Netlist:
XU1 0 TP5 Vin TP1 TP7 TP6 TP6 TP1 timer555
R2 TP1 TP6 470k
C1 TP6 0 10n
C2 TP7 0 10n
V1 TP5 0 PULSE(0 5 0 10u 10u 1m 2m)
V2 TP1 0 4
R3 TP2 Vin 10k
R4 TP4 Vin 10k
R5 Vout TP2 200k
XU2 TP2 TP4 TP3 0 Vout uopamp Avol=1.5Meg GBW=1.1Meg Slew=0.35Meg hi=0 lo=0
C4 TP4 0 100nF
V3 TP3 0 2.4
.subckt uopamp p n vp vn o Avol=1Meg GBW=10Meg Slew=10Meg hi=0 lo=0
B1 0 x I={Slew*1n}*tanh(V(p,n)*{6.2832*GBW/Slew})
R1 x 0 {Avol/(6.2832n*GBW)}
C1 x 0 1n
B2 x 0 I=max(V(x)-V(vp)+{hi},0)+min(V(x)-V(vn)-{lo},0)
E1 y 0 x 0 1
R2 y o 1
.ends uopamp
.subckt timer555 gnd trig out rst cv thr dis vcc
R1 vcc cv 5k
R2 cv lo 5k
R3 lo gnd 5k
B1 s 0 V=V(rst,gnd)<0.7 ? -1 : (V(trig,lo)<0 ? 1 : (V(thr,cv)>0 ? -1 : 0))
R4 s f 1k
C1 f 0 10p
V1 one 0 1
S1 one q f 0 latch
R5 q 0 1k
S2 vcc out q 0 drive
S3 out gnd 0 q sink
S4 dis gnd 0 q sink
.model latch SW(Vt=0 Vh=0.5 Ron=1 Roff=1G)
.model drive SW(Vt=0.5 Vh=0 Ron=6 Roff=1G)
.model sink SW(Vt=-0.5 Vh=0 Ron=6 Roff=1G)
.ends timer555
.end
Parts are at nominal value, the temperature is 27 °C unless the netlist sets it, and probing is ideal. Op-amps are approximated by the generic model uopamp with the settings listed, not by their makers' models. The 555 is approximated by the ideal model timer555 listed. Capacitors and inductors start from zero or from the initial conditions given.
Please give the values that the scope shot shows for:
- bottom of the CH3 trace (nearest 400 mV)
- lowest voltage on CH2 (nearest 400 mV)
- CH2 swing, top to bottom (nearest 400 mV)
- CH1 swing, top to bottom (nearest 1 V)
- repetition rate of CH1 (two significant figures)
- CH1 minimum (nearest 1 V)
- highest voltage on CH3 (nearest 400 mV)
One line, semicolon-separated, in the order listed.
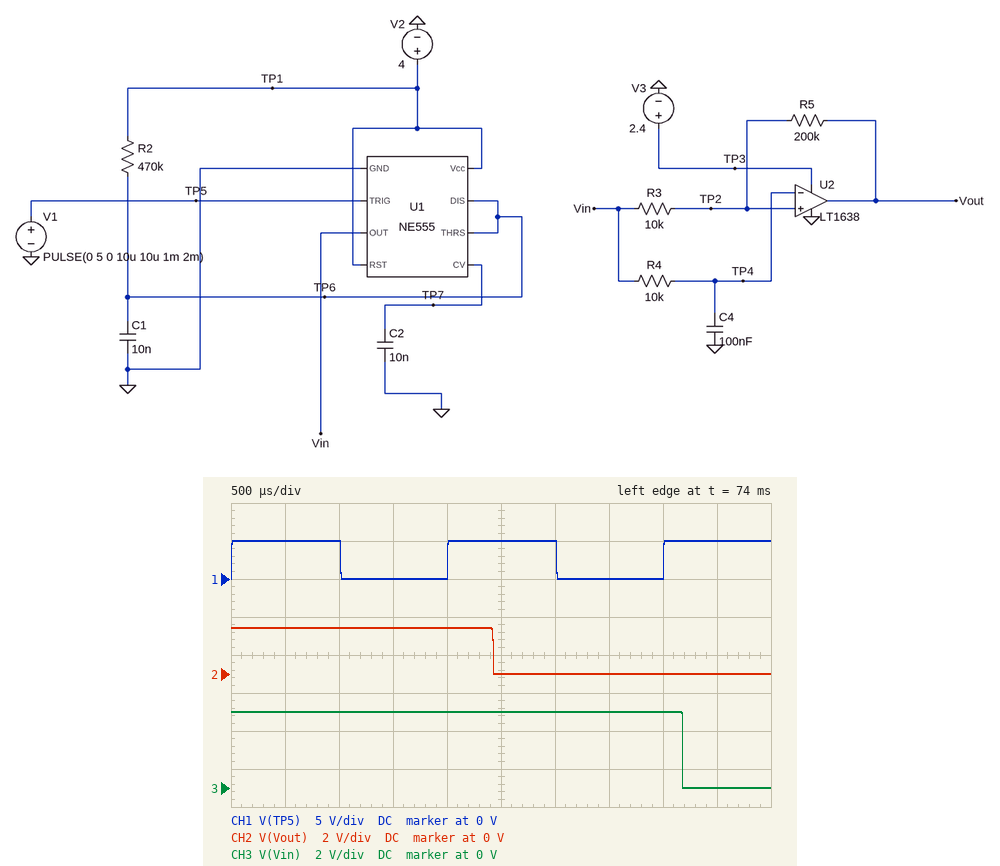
0 V; 0 V; 2.4 V; 5 V; 500 Hz; 0 V; 4.0 V
